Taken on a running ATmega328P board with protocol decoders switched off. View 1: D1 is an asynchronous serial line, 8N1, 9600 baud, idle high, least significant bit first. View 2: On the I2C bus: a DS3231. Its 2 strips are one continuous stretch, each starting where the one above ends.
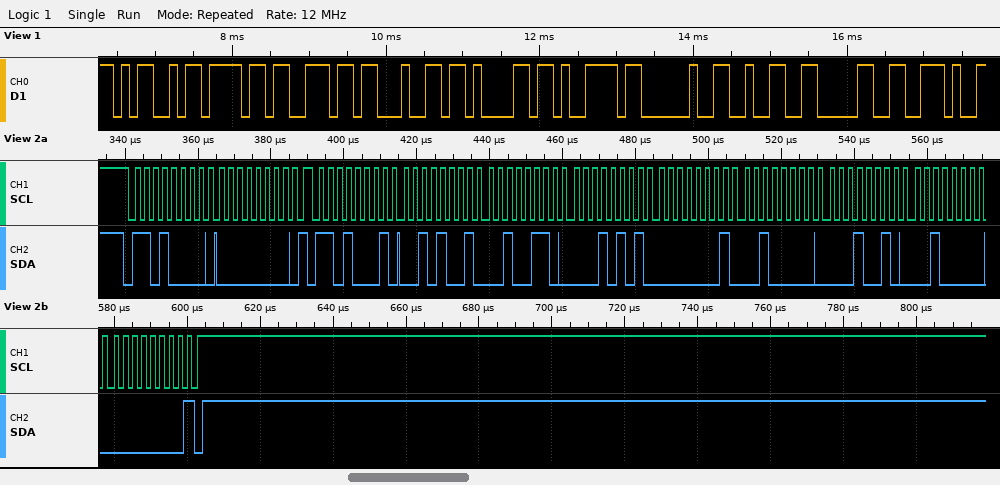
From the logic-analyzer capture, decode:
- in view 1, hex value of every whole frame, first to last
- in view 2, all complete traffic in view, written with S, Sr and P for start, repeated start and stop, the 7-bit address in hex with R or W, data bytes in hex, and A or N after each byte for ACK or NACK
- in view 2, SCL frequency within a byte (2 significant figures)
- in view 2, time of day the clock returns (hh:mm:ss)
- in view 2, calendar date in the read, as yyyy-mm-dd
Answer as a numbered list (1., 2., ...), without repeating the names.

1. 4D 6F 6E 64 61 79 20 32 30 2E
2. S 68W A 00 A Sr 68R A 29 A 26 A 15 A 01 A 20 A 12 A 20 A 00 N P
3. 400 kHz
4. 15:26:29
5. 2020-12-20
